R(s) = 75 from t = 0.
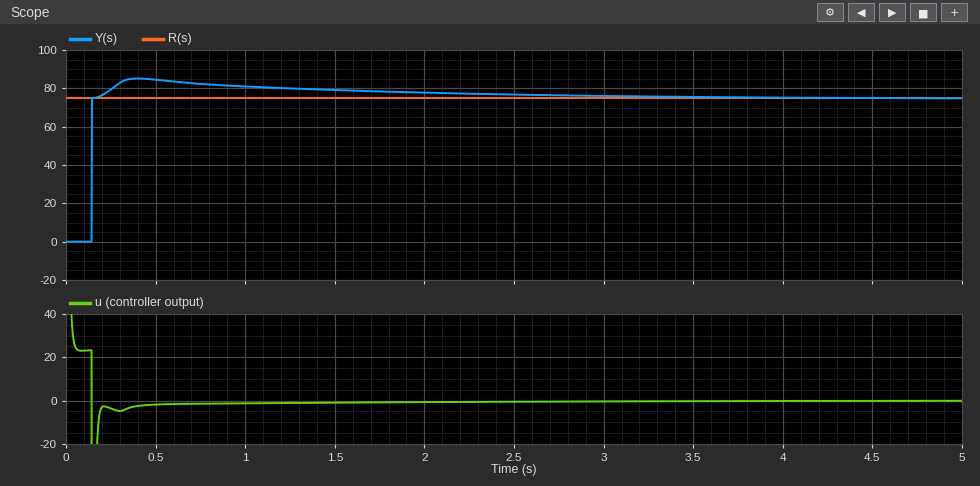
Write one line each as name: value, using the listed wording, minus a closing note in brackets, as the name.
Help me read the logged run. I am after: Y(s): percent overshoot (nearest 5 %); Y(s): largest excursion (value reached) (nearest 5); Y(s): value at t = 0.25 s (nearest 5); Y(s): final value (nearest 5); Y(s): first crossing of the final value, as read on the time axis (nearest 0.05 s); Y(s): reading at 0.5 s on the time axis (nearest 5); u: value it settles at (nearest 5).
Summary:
Y(s): percent overshoot: 15 %
Y(s): largest excursion (value reached): 85
Y(s): value at t = 0.25 s: 80
Y(s): final value: 75
Y(s): first crossing of the final value, as read on the time axis: 0.15 s
Y(s): reading at 0.5 s on the time axis: 85
u: value it settles at: 0
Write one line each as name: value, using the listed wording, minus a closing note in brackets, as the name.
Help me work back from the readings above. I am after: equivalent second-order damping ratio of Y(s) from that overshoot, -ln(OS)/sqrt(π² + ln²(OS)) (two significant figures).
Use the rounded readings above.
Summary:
equivalent second-order damping ratio of Y(s) from that overshoot, -ln(OS)/sqrt(π² + ln²(OS)): 0.52
